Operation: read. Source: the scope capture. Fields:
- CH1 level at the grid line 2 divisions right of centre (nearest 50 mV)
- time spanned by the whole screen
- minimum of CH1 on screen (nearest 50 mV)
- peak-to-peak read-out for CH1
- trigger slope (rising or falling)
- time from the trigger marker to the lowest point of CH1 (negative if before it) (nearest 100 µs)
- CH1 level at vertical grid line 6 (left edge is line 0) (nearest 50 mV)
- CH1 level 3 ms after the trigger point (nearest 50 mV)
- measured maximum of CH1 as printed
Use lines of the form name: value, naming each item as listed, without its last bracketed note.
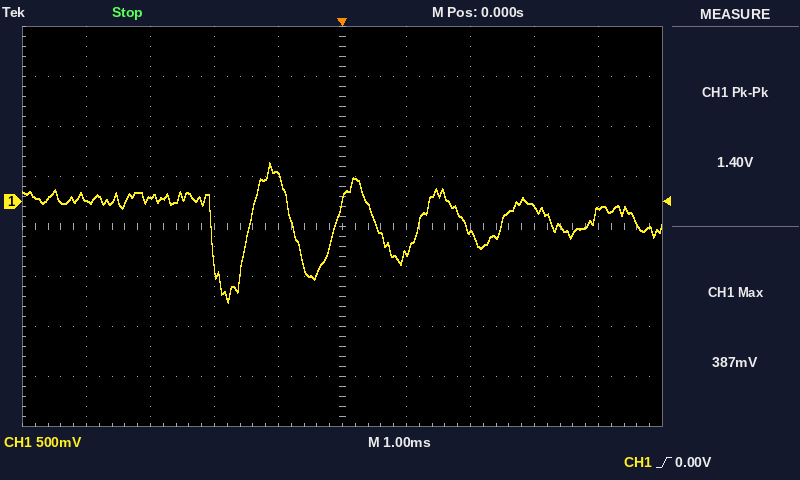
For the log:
CH1 level at the grid line 2 divisions right of centre: -300 mV
time spanned by the whole screen: 10 ms
minimum of CH1 on screen: -1.00 V
peak-to-peak read-out for CH1: 1.40 V
trigger slope: rising
time from the trigger marker to the lowest point of CH1 (negative if before it): -1.8 ms
CH1 level at vertical grid line 6 (left edge is line 0): -500 mV
CH1 level 3 ms after the trigger point: -50 mV
measured maximum of CH1 as printed: 387 mV
